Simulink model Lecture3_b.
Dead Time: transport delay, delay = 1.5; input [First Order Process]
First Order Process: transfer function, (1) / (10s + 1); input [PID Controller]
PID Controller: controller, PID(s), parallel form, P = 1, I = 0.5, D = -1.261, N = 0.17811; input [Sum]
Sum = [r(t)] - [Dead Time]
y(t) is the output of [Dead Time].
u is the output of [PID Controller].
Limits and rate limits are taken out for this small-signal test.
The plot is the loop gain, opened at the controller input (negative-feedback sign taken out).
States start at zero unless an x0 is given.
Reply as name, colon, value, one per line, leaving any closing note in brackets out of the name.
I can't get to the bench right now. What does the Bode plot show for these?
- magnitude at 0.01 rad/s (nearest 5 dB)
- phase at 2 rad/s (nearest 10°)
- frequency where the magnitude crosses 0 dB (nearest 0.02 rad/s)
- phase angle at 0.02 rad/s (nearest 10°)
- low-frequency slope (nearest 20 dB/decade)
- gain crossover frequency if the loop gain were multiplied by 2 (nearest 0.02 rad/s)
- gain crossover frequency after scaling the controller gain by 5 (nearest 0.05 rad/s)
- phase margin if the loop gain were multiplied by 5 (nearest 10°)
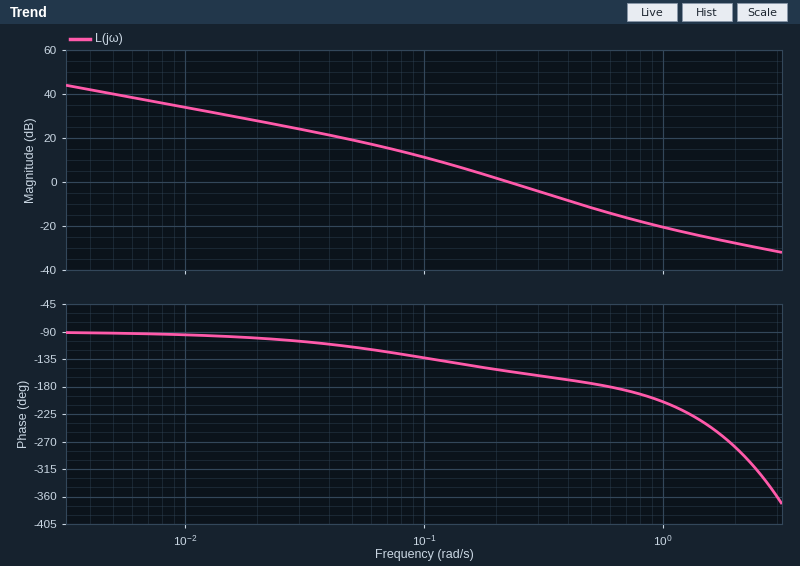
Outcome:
magnitude at 0.01 rad/s: 35 dB
phase at 2 rad/s: -280°
frequency where the magnitude crosses 0 dB: 0.22 rad/s
phase angle at 0.02 rad/s: -100°
low-frequency slope: -20 dB/decade
gain crossover frequency if the loop gain were multiplied by 2: 0.34 rad/s
gain crossover frequency after scaling the controller gain by 5: 0.60 rad/s
phase margin if the loop gain were multiplied by 5: 0°
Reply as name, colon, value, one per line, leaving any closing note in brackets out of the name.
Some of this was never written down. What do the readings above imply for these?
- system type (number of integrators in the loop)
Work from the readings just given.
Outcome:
system type: 1
